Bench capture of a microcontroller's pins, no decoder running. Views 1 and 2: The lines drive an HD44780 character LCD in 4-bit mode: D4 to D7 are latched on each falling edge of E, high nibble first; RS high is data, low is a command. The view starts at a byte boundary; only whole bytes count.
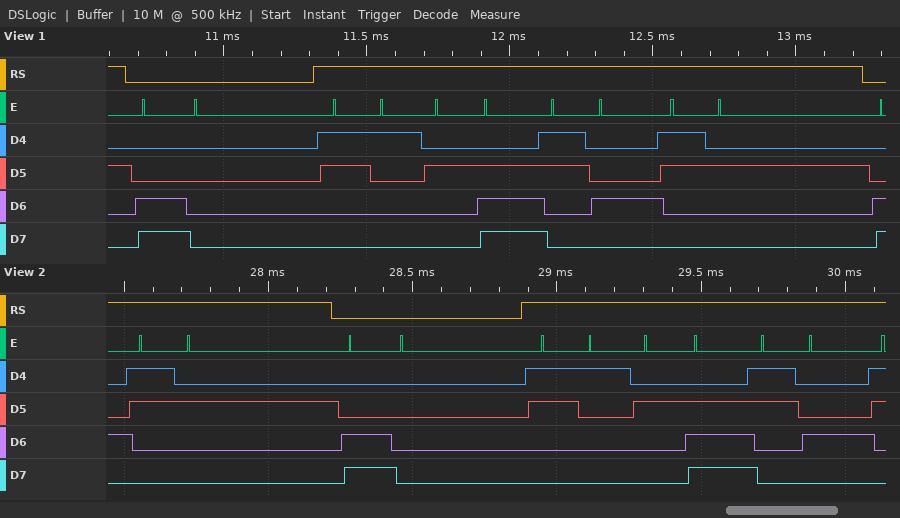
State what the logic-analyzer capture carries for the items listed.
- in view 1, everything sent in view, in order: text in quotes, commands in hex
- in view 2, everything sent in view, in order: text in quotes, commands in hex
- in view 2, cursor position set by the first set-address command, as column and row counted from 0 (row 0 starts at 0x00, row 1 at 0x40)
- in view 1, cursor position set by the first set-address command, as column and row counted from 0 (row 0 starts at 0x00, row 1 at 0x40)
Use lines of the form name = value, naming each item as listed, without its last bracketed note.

in view 1, everything sent in view, in order: text in quotes, commands in hex = 0xC0 "1.42"
in view 2, everything sent in view, in order: text in quotes, commands in hex = "2" 0xC0 "1.4"
in view 2, cursor position set by the first set-address command, as column and row counted from 0 = column 0, row 1
in view 1, cursor position set by the first set-address command, as column and row counted from 0 = column 0, row 1
